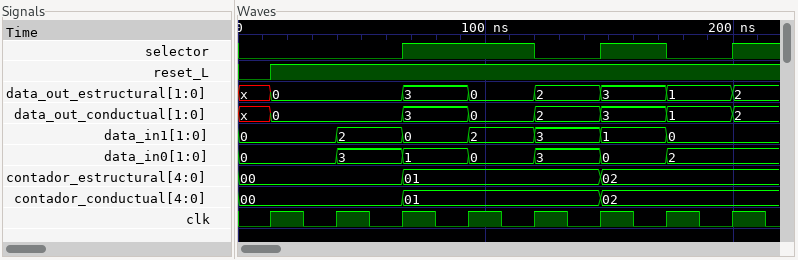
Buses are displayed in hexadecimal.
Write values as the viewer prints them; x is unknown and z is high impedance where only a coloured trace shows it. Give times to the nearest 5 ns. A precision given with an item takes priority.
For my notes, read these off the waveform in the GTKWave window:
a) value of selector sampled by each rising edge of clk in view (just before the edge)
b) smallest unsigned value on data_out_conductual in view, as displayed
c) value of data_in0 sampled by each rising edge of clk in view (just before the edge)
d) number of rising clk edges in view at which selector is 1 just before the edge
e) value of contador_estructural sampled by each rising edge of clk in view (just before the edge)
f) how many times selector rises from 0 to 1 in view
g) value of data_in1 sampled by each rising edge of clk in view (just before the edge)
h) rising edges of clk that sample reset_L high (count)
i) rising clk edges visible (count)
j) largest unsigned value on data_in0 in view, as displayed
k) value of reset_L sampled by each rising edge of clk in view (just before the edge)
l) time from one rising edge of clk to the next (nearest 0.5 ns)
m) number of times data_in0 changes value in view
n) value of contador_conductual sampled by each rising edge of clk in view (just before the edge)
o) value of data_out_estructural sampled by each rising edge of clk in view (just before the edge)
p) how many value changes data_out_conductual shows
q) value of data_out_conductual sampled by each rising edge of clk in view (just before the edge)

0 0 0 1 1 0 1 0
0
0, 0, 3, 1, 0, 3, 0, 2
3
00, 00, 00, 01, 01, 01, 02, 02
3
0, 0, 2, 0, 2, 3, 1, 0
7
8
3
0 1 1 1 1 1 1 1
26.5 ns
6
00, 00, 00, 01, 01, 01, 02, 02
x, 0, 0, 3, 0, 2, 3, 1
7
x, 0, 0, 3, 0, 2, 3, 1
